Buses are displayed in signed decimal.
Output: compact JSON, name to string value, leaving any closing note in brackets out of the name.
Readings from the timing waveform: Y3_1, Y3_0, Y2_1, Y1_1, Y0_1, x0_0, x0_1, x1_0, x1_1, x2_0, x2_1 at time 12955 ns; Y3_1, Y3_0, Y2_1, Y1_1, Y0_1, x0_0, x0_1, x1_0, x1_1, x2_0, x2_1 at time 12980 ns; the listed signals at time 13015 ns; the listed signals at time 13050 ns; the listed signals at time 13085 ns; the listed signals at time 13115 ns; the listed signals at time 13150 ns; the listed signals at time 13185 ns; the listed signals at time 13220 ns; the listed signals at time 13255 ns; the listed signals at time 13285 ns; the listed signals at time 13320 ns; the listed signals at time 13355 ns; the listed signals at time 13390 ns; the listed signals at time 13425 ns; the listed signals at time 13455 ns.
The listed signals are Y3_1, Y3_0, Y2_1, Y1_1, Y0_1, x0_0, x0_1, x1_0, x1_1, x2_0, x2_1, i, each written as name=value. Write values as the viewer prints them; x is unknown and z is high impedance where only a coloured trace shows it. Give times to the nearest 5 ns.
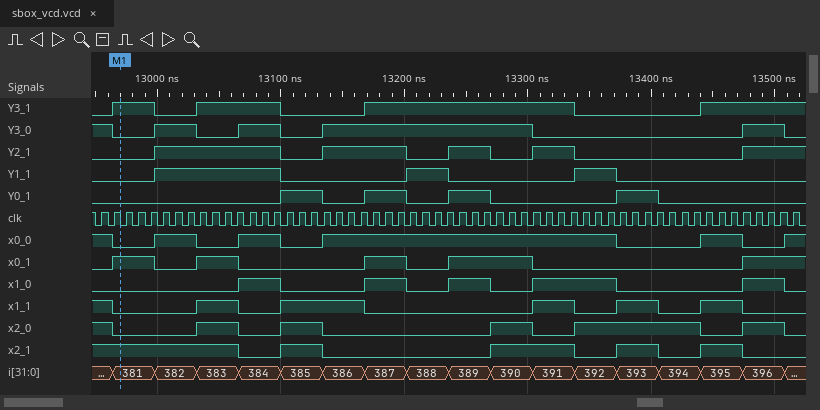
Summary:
{"Y3_1, Y3_0, Y2_1, Y1_1, Y0_1, x0_0, x0_1, x1_0, x1_1, x2_0, x2_1 at time 12955 ns": "Y3_1=0, Y3_0=1, Y2_1=0, Y1_1=0, Y0_1=0, x0_0=1, x0_1=0, x1_0=0, x1_1=1, x2_0=1, x2_1=1", "Y3_1, Y3_0, Y2_1, Y1_1, Y0_1, x0_0, x0_1, x1_0, x1_1, x2_0, x2_1 at time 12980 ns": "Y3_1=1, Y3_0=0, Y2_1=0, Y1_1=0, Y0_1=0, x0_0=0, x0_1=1, x1_0=0, x1_1=0, x2_0=0, x2_1=1", "the listed signals at time 13015 ns": "Y3_1=0, Y3_0=1, Y2_1=1, Y1_1=1, Y0_1=0, x0_0=1, x0_1=0, x1_0=0, x1_1=0, x2_0=0, x2_1=1, i=382", "the listed signals at time 13050 ns": "Y3_1=1, Y3_0=0, Y2_1=1, Y1_1=1, Y0_1=0, x0_0=0, x0_1=1, x1_0=0, x1_1=1, x2_0=1, x2_1=1, i=383", "the listed signals at time 13085 ns": "Y3_1=1, Y3_0=1, Y2_1=1, Y1_1=1, Y0_1=0, x0_0=1, x0_1=0, x1_0=1, x1_1=0, x2_0=0, x2_1=0, i=384", "the listed signals at time 13115 ns": "Y3_1=0, Y3_0=0, Y2_1=0, Y1_1=0, Y0_1=1, x0_0=0, x0_1=0, x1_0=0, x1_1=1, x2_0=1, x2_1=1, i=385", "the listed signals at time 13150 ns": "Y3_1=0, Y3_0=1, Y2_1=1, Y1_1=0, Y0_1=0, x0_0=1, x0_1=0, x1_0=0, x1_1=1, x2_0=0, x2_1=0, i=386", "the listed signals at time 13185 ns": "Y3_1=1, Y3_0=1, Y2_1=1, Y1_1=0, Y0_1=1, x0_0=1, x0_1=1, x1_0=1, x1_1=0, x2_0=0, x2_1=0, i=387", "the listed signals at time 13220 ns": "Y3_1=1, Y3_0=1, Y2_1=0, Y1_1=1, Y0_1=0, x0_0=1, x0_1=0, x1_0=0, x1_1=0, x2_0=0, x2_1=0, i=388", "the listed signals at time 13255 ns": "Y3_1=1, Y3_0=1, Y2_1=1, Y1_1=0, Y0_1=1, x0_0=1, x0_1=1, x1_0=1, x1_1=0, x2_0=0, x2_1=0, i=389", "the listed signals at time 13285 ns": "Y3_1=1, Y3_0=1, Y2_1=0, Y1_1=0, Y0_1=0, x0_0=1, x0_1=1, x1_0=0, x1_1=0, x2_0=1, x2_1=1, i=390", "the listed signals at time 13320 ns": "Y3_1=1, Y3_0=0, Y2_1=1, Y1_1=0, Y0_1=0, x0_0=1, x0_1=0, x1_0=1, x1_1=1, x2_0=0, x2_1=1, i=391", "the listed signals at time 13355 ns": "Y3_1=0, Y3_0=0, Y2_1=0, Y1_1=1, Y0_1=0, x0_0=1, x0_1=0, x1_0=1, x1_1=0, x2_0=1, x2_1=0, i=392", "the listed signals at time 13390 ns": "Y3_1=0, Y3_0=0, Y2_1=0, Y1_1=0, Y0_1=1, x0_0=0, x0_1=0, x1_0=0, x1_1=1, x2_0=1, x2_1=1, i=393", "the listed signals at time 13425 ns": "Y3_1=0, Y3_0=0, Y2_1=0, Y1_1=0, Y0_1=0, x0_0=0, x0_1=0, x1_0=0, x1_1=0, x2_0=1, x2_1=0, i=394", "the listed signals at time 13455 ns": "Y3_1=1, Y3_0=0, Y2_1=0, Y1_1=0, Y0_1=0, x0_0=1, x0_1=0, x1_0=0, x1_1=1, x2_0=0, x2_1=1, i=395"}
